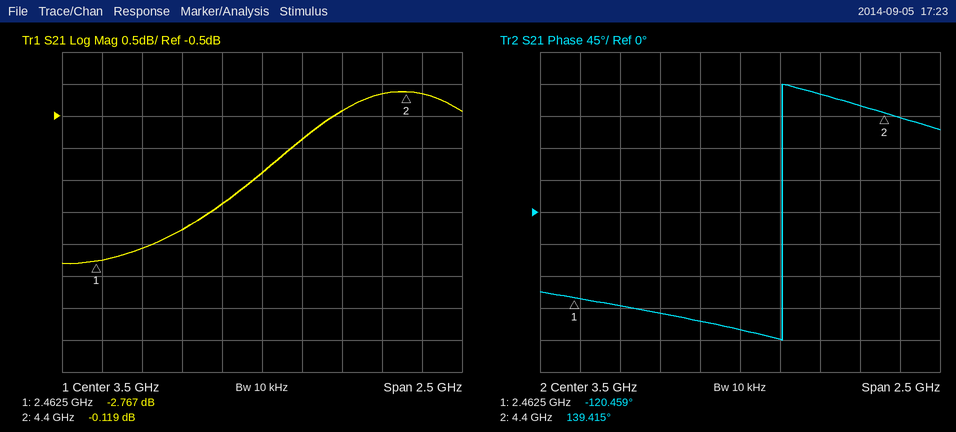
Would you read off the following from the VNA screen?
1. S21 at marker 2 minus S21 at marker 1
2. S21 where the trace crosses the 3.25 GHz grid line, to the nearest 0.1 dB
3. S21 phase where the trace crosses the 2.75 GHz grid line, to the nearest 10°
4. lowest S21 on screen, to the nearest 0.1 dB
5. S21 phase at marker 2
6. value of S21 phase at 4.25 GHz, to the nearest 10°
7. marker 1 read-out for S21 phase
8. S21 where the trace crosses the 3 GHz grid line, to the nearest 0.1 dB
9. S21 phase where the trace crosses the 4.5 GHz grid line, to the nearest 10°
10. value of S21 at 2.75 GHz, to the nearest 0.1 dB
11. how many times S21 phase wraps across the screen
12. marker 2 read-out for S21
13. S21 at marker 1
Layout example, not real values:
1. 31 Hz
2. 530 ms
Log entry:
1. 2.648 dB
2. -1.9 dB
3. -130°
4. -2.8 dB
5. 139.415°
6. 150°
7. -120.459°
8. -2.3 dB
9. 130°
10. -2.6 dB
11. 1
12. -0.119 dB
13. -2.767 dB
